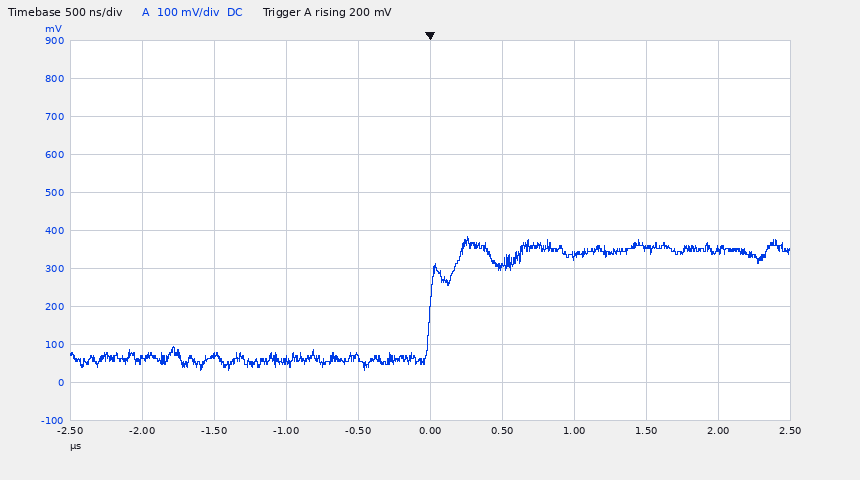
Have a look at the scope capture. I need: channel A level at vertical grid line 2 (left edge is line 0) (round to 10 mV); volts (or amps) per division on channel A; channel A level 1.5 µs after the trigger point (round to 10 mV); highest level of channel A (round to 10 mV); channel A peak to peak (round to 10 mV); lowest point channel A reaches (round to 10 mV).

70 mV
100 mV
350 mV
380 mV
350 mV
30 mV
